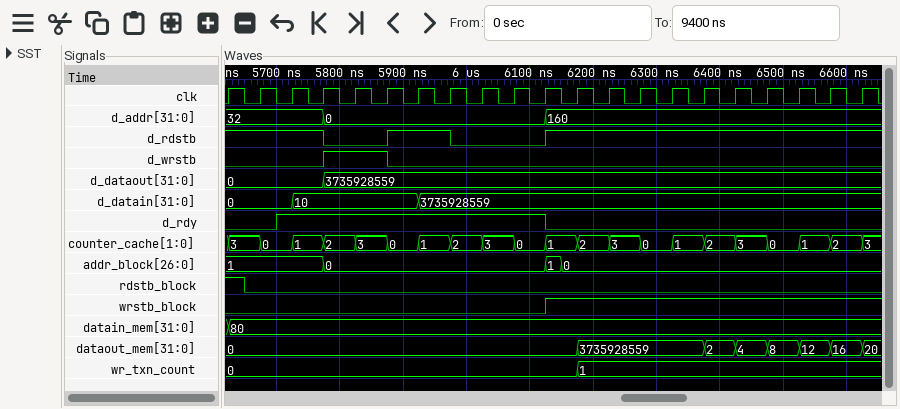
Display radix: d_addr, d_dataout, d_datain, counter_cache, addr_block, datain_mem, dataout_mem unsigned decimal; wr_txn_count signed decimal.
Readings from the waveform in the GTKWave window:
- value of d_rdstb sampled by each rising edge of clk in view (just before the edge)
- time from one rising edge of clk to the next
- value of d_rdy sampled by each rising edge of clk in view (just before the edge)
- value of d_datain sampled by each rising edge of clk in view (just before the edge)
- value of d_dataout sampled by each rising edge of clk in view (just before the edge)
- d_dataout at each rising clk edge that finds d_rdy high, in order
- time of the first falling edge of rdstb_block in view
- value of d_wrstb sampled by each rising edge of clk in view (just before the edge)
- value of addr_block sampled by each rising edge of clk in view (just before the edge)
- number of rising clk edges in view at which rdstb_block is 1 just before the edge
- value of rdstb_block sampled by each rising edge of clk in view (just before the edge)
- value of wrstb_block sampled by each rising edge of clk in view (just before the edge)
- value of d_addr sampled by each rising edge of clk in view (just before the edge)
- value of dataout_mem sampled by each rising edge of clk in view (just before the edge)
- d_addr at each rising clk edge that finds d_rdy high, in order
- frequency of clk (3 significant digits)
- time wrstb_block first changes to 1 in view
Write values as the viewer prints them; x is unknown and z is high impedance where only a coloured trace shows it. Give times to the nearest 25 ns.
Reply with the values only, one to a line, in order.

1 1 1 1 0 0 1 1 0 0 0 1 1 1 1 1 1 1 1 1 1
50 ns
0 0 1 1 1 1 1 1 1 1 1 0 0 0 0 0 0 0 0 0 0
0, 0, 0, 10, 10, 10, 10, 3735928559, 3735928559, 3735928559, 3735928559, 3735928559, 3735928559, 3735928559, 3735928559, 3735928559, 3735928559, 3735928559, 3735928559, 3735928559, 3735928559
0, 0, 0, 0, 3735928559, 3735928559, 3735928559, 3735928559, 3735928559, 3735928559, 3735928559, 3735928559, 3735928559, 3735928559, 3735928559, 3735928559, 3735928559, 3735928559, 3735928559, 3735928559, 3735928559
0, 0, 3735928559, 3735928559, 3735928559, 3735928559, 3735928559, 3735928559, 3735928559
5650 ns
0 0 0 0 1 1 0 0 0 0 0 0 0 0 0 0 0 0 0 0 0
1, 1, 1, 1, 0, 0, 0, 0, 0, 0, 0, 0, 0, 0, 0, 0, 0, 0, 0, 0, 0
1
1 0 0 0 0 0 0 0 0 0 0 0 0 0 0 0 0 0 0 0 0
0 0 0 0 0 0 0 0 0 0 0 1 1 1 1 1 1 1 1 1 1
32, 32, 32, 32, 0, 0, 0, 0, 0, 0, 0, 160, 160, 160, 160, 160, 160, 160, 160, 160, 160
0, 0, 0, 0, 0, 0, 0, 0, 0, 0, 0, 0, 3735928559, 3735928559, 3735928559, 3735928559, 2, 4, 8, 12, 16
32, 32, 0, 0, 0, 0, 0, 0, 0
20.0 MHz
6125 ns
